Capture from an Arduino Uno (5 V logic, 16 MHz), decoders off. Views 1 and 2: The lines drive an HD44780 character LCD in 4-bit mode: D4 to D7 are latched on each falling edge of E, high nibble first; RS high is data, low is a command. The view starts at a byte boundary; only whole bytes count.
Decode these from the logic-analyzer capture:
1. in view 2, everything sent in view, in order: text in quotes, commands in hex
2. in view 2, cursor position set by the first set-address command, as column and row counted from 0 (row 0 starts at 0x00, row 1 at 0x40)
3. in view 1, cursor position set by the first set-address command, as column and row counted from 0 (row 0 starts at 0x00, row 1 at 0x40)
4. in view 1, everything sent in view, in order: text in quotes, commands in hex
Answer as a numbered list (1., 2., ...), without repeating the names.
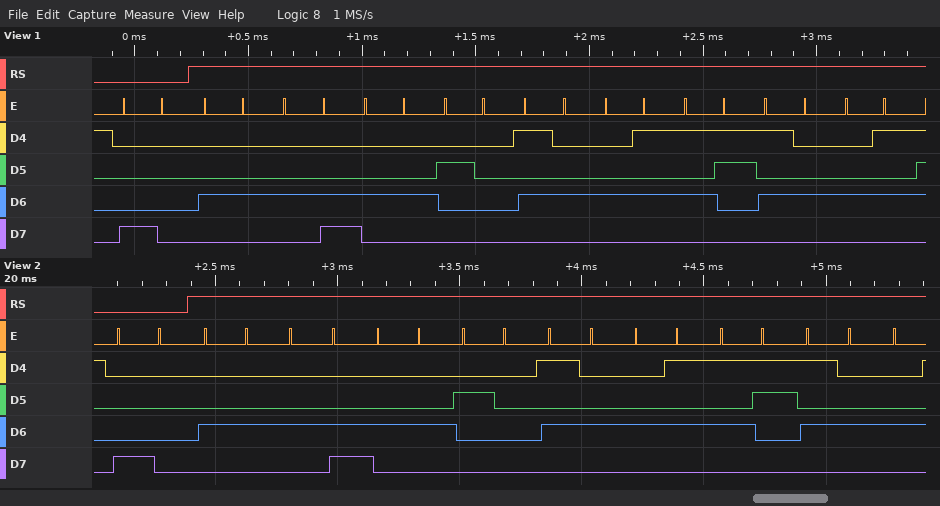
1. 0x80 "DLD TEST"
2. column 0, row 0
3. column 0, row 0
4. 0x80 "DLD TESTE"
